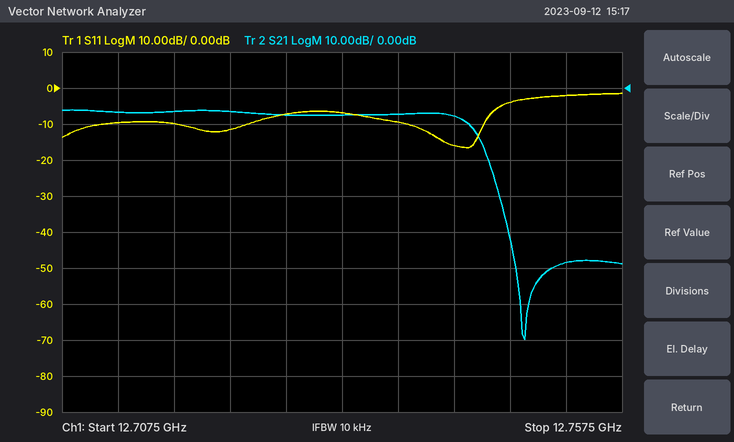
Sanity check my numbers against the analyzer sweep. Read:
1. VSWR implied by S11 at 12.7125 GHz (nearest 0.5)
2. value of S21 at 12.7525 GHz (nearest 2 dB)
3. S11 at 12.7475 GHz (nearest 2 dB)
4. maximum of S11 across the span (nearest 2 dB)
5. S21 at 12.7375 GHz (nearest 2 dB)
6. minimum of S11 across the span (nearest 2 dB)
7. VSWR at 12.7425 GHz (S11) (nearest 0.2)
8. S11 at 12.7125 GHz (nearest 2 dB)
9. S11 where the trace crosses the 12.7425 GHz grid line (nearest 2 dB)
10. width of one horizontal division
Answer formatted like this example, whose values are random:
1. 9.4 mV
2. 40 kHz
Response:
1. 2.0
2. -48 dB
3. -4 dB
4. -2 dB
5. -8 dB
6. -16 dB
7. 1.4
8. -10 dB
9. -16 dB
10. 5 MHz
